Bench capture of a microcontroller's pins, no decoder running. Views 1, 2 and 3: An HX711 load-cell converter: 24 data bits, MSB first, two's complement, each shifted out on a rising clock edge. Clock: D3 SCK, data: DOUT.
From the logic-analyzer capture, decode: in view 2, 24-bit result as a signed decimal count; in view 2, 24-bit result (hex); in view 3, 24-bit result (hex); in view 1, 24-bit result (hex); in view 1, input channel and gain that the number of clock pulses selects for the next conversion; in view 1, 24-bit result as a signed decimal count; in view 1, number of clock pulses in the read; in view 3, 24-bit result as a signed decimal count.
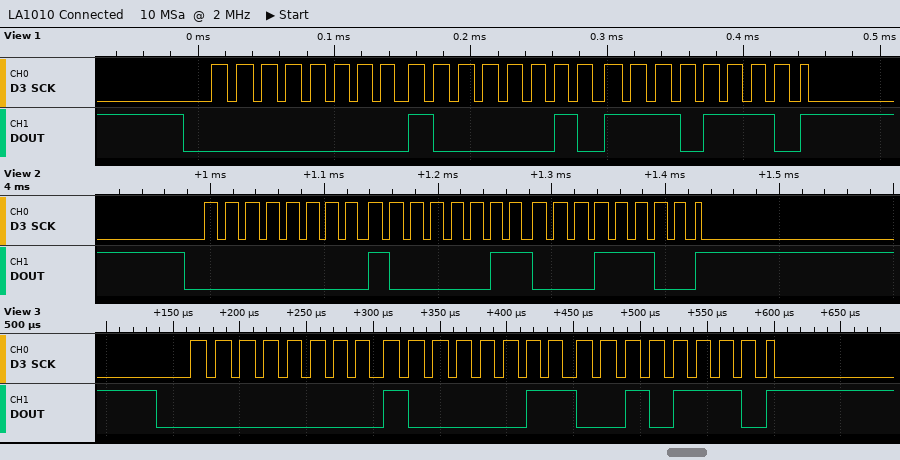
33564
0x00831C
0x00832E
0x0082EE
channel A, gain 128
33518
25
33582
